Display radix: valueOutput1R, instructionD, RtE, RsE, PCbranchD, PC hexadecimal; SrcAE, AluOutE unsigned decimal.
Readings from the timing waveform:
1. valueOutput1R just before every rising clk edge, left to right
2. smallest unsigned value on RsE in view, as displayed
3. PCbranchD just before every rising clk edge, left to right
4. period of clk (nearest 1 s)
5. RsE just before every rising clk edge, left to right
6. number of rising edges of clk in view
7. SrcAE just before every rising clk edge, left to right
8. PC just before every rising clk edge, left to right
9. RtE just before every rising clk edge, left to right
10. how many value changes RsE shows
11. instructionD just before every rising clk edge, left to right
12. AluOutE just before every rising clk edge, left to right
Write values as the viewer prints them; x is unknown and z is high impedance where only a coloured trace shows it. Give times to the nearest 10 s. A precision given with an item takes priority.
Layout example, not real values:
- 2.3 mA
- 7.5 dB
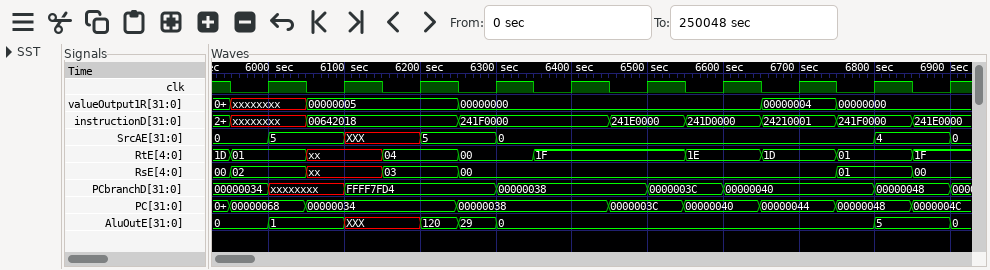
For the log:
- xxxxxxxx, 00000005, 00000005, 00000000, 00000000, 00000000, 00000000, 00000004, 00000000, 00000000
- 00
- 00000034, xxxxxxxx, FFFF7FD4, FFFF7FD4, 00000038, 00000038, 0000003C, 00000040, 00000040, 00000048
- 100 s
- 02, xx, 03, 00, 00, 00, 00, 00, 01, 00
- 10
- 0, 5, XXX, 5, 0, 0, 0, 0, 0, 4
- 00000068, 00000034, 00000034, 00000038, 00000038, 0000003C, 00000040, 00000044, 00000048, 0000004C
- 01, xx, 04, 00, 1F, 1F, 1E, 1D, 01, 1F
- 6
- xxxxxxxx, 00642018, 00642018, 241F0000, 241F0000, 241E0000, 241D0000, 24210001, 241F0000, 241E0000
- 0, 1, XXX, 29, 0, 0, 0, 0, 0, 5
